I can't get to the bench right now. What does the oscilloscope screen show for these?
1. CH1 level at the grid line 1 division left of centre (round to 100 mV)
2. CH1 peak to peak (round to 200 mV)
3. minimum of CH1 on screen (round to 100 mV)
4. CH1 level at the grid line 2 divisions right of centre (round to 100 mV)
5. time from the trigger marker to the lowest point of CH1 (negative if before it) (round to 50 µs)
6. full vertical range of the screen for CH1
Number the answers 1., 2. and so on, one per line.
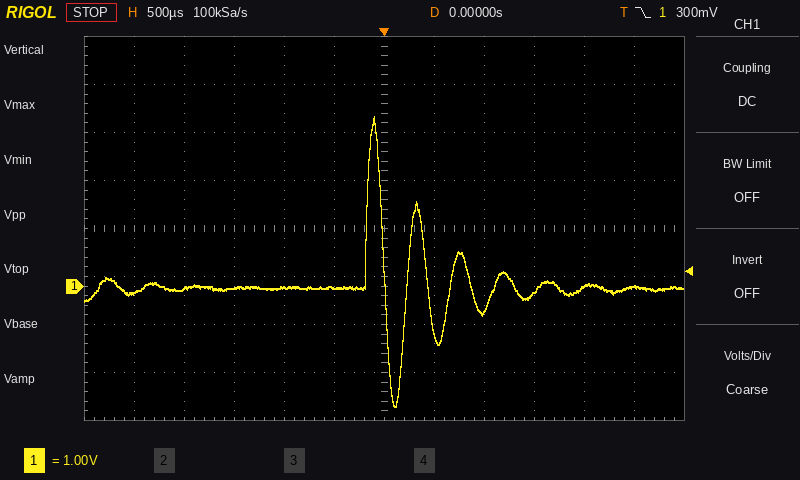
1. 0.0 V
2. 6.0 V
3. -2.5 V
4. -500 mV
5. +100 µs
6. 8 V
